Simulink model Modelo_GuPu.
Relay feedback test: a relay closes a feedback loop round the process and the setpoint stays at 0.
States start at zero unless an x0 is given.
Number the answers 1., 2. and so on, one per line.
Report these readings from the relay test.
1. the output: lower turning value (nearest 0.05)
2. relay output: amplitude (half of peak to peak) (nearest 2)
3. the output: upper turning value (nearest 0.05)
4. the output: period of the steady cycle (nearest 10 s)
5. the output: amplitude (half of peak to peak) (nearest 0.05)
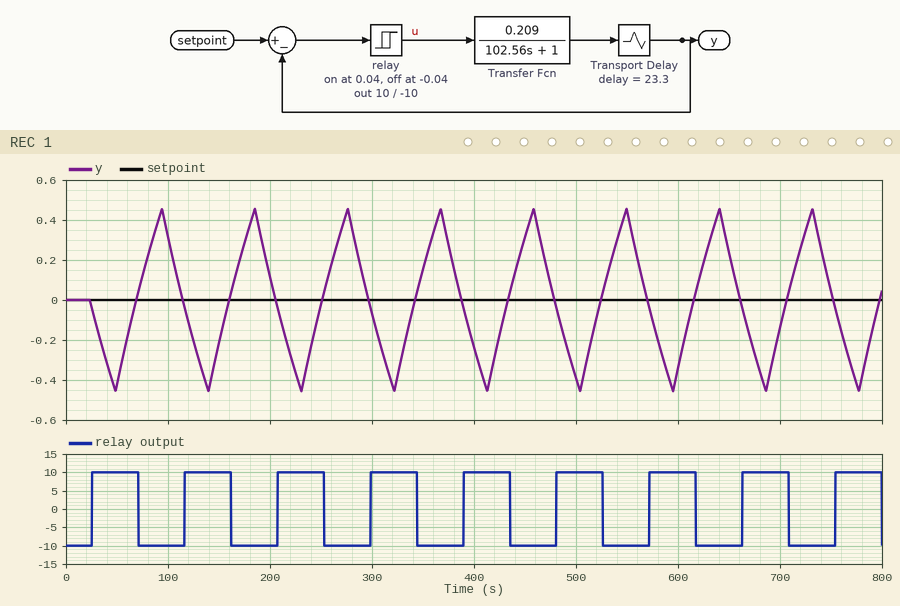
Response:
1. -0.45
2. 10
3. 0.45
4. 90 s
5. 0.45
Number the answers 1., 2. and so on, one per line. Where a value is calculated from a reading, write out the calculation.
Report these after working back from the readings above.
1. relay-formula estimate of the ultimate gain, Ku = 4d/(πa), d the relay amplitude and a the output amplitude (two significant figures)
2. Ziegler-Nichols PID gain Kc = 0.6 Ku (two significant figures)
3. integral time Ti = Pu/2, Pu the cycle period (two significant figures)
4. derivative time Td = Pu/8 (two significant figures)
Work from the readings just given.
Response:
1. 4 × 10 / (π × 0.45) = 28
2. 0.6 × 28 = 17
3. 90 / 2 = 45 s
4. 90 / 8 = 11 s
